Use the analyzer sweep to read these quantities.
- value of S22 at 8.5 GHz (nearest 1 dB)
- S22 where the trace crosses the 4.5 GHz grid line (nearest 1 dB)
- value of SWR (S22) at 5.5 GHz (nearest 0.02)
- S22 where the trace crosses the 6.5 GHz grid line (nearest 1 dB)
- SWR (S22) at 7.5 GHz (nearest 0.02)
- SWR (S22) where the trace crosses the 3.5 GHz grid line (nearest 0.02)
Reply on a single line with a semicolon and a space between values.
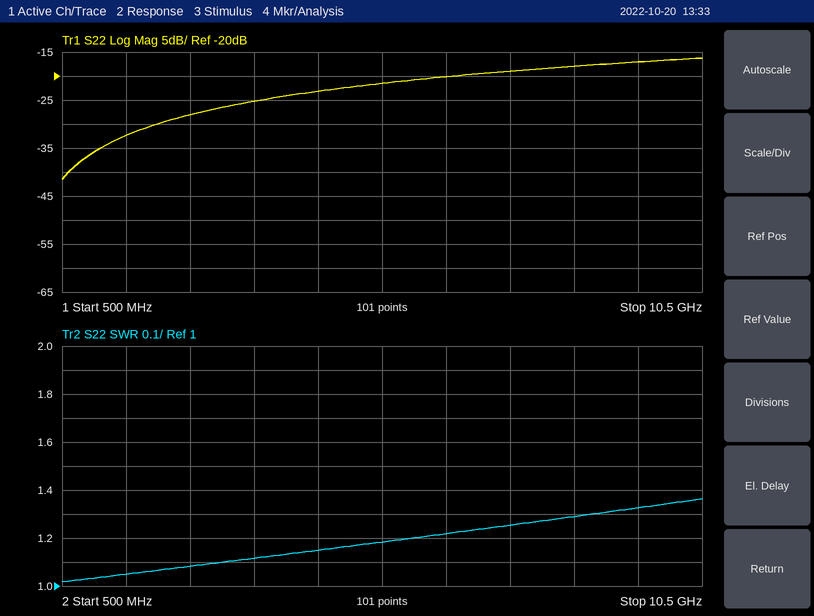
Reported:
-18 dB; -23 dB; 1.18; -20 dB; 1.26; 1.12
